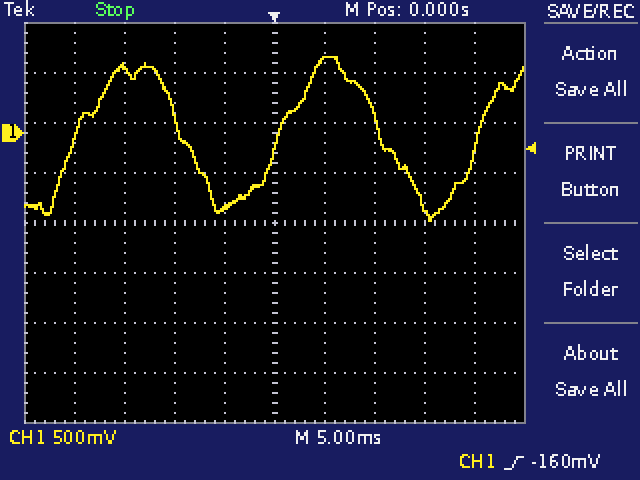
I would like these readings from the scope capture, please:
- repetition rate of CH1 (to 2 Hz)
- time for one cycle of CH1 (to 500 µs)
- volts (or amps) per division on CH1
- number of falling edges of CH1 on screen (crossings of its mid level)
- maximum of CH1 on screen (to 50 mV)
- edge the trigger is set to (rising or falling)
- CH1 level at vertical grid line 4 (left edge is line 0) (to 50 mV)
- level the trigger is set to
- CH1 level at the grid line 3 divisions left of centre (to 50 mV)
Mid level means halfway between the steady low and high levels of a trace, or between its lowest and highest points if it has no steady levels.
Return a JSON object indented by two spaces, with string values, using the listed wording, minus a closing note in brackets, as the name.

{
  "repetition rate of CH1": "50 Hz",
  "time for one cycle of CH1": "20.0 ms",
  "volts (or amps) per division on CH1": "500 mV",
  "number of falling edges of CH1 on screen": "2",
  "maximum of CH1 on screen": "750 mV",
  "edge the trigger is set to": "rising",
  "CH1 level at vertical grid line 4 (left edge is line 0)": "-750 mV",
  "level the trigger is set to": "-160 mV",
  "CH1 level at the grid line 3 divisions left of centre": "650 mV"
}
